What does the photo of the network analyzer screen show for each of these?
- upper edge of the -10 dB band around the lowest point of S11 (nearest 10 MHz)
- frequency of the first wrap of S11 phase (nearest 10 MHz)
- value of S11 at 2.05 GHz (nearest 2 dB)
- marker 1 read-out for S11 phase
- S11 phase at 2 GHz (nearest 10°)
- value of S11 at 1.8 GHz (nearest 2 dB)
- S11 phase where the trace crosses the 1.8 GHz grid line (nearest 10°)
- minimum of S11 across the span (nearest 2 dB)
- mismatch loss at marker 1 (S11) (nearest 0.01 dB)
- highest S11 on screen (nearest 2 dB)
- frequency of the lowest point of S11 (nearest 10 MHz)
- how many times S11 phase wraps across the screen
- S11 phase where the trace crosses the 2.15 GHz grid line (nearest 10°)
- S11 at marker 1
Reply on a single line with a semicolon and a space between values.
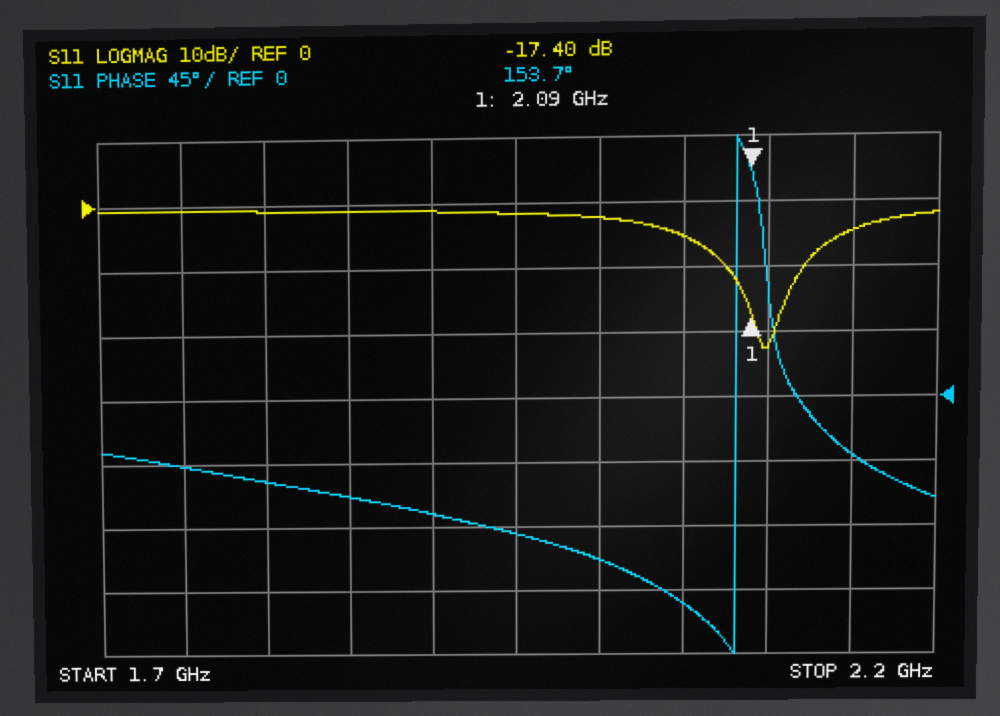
2.12 GHz; 2.08 GHz; -6 dB; 153.7°; -110°; 0 dB; -60°; -22 dB; 0.08 dB; 0 dB; 2.10 GHz; 1; -40°; -17.40 dB
